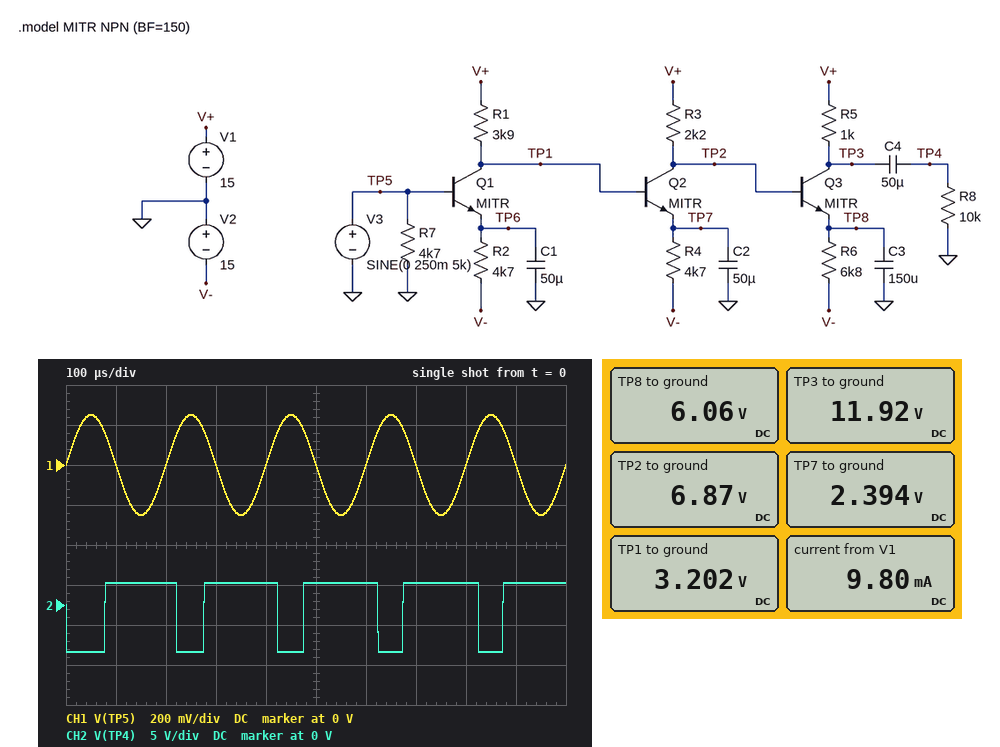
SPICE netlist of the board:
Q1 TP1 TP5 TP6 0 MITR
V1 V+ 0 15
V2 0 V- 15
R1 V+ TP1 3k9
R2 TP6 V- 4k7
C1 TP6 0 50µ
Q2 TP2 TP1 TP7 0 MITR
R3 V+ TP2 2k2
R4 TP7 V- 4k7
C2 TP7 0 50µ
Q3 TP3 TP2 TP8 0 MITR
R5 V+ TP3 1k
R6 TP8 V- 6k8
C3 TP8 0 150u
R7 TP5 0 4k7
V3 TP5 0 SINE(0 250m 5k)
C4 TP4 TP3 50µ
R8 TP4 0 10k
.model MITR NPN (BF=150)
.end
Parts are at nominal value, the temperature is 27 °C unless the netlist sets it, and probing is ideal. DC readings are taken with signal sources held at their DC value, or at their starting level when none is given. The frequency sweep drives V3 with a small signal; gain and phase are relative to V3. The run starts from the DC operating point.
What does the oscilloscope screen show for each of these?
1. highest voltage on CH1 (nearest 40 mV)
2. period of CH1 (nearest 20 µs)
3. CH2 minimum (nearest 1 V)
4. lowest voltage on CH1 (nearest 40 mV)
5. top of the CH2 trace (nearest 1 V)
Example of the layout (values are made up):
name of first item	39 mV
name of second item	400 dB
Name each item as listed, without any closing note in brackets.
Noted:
highest voltage on CH1	240 mV
period of CH1	200 µs
CH2 minimum	-6 V
lowest voltage on CH1	-240 mV
top of the CH2 trace	3 V
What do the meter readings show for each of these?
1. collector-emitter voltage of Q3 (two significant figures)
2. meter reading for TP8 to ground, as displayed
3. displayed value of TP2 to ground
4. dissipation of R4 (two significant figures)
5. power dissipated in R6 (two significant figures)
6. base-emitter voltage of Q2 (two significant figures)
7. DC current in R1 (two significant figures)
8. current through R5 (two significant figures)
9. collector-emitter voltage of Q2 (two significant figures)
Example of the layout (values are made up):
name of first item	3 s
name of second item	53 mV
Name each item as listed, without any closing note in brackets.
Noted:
collector-emitter voltage of Q3	5.9 V
meter reading for TP8 to ground, as displayed	6.06 V
displayed value of TP2 to ground	6.87 V
dissipation of R4	64 mW
power dissipated in R6	65 mW
base-emitter voltage of Q2	810 mV
DC current in R1	3.0 mA
current through R5	3.1 mA
collector-emitter voltage of Q2	4.5 V
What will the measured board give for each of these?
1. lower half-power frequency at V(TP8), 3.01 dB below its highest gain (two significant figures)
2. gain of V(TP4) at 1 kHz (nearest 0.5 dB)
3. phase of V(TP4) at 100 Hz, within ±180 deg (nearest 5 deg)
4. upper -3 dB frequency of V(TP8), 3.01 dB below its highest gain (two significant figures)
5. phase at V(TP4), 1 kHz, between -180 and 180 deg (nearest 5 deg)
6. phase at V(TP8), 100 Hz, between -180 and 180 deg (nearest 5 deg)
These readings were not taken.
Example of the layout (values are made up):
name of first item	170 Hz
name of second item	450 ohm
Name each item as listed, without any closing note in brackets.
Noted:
lower half-power frequency at V(TP8), 3.01 dB below its highest gain	82 Hz
gain of V(TP4) at 1 kHz	121.0 dB
phase of V(TP4) at 100 Hz, within ±180 deg	-35 deg
upper -3 dB frequency of V(TP8), 3.01 dB below its highest gain	560 Hz
phase at V(TP4), 1 kHz, between -180 and 180 deg	-150 deg
phase at V(TP8), 100 Hz, between -180 and 180 deg	55 deg
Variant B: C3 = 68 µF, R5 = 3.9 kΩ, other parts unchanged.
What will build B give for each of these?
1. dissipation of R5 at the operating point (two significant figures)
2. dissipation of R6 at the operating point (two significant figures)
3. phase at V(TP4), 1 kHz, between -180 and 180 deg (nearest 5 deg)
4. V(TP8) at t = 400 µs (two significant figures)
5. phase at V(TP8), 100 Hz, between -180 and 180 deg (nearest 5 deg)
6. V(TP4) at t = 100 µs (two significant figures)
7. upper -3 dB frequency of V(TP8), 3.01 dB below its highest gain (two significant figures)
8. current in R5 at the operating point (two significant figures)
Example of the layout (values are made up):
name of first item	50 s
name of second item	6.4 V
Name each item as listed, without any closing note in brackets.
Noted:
dissipation of R5 at the operating point	25 mW
dissipation of R6 at the operating point	60 mW
phase at V(TP4), 1 kHz, between -180 and 180 deg	-150 deg
V(TP8) at t = 400 µs	5.1 V
phase at V(TP8), 100 Hz, between -180 and 180 deg	30 deg
V(TP4) at t = 100 µs	7.1 V
upper -3 dB frequency of V(TP8), 3.01 dB below its highest gain	540 Hz
current in R5 at the operating point	2.5 mA
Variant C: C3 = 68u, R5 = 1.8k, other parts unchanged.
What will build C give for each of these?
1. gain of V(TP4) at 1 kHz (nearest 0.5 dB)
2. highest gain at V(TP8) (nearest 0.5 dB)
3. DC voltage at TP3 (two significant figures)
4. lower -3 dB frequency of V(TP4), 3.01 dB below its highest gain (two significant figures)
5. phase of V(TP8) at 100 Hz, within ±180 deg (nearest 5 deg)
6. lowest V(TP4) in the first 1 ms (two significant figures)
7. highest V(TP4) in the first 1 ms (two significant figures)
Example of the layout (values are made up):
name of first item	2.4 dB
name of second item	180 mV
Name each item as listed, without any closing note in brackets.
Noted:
gain of V(TP4) at 1 kHz	125.5 dB
highest gain at V(TP8)	75.5 dB
DC voltage at TP3	9.5 V
lower -3 dB frequency of V(TP4), 3.01 dB below its highest gain	420 Hz
phase of V(TP8) at 100 Hz, within ±180 deg	75 deg
lowest V(TP4) in the first 1 ms	-3.4 V
highest V(TP4) in the first 1 ms	4.7 V
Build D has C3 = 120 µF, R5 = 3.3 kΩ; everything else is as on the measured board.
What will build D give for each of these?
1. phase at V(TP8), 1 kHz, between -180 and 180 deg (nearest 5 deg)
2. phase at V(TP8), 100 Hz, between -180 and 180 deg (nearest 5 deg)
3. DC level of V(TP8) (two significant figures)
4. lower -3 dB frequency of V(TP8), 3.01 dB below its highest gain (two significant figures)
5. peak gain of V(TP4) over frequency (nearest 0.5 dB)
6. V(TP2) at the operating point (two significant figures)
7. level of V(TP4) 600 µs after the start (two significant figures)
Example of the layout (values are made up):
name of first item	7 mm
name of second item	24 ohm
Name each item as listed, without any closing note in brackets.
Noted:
phase at V(TP8), 1 kHz, between -180 and 180 deg	-65 deg
phase at V(TP8), 100 Hz, between -180 and 180 deg	30 deg
DC level of V(TP8)	5.6 V
lower -3 dB frequency of V(TP8), 3.01 dB below its highest gain	68 Hz
peak gain of V(TP4) over frequency	64.0 dB
V(TP2) at the operating point	6.4 V
level of V(TP4) 600 µs after the start	7.0 V
